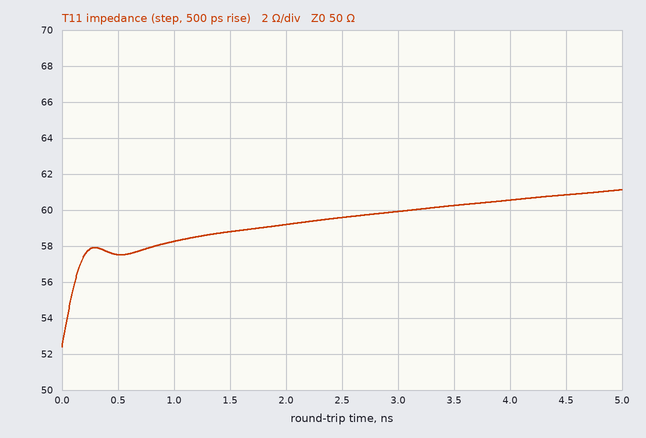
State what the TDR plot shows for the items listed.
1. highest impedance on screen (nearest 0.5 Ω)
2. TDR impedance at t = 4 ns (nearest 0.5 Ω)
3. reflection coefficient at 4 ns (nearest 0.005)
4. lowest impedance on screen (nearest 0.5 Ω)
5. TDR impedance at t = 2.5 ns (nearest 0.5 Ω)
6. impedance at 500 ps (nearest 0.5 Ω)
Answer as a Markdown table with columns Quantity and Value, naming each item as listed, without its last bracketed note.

| Quantity | Value |
|---|---|
| highest impedance on screen | 61.0 Ω |
| TDR impedance at t = 4 ns | 60.5 Ω |
| reflection coefficient at 4 ns | +0.095 |
| lowest impedance on screen | 52.5 Ω |
| TDR impedance at t = 2.5 ns | 59.5 Ω |
| impedance at 500 ps | 57.5 Ω |
